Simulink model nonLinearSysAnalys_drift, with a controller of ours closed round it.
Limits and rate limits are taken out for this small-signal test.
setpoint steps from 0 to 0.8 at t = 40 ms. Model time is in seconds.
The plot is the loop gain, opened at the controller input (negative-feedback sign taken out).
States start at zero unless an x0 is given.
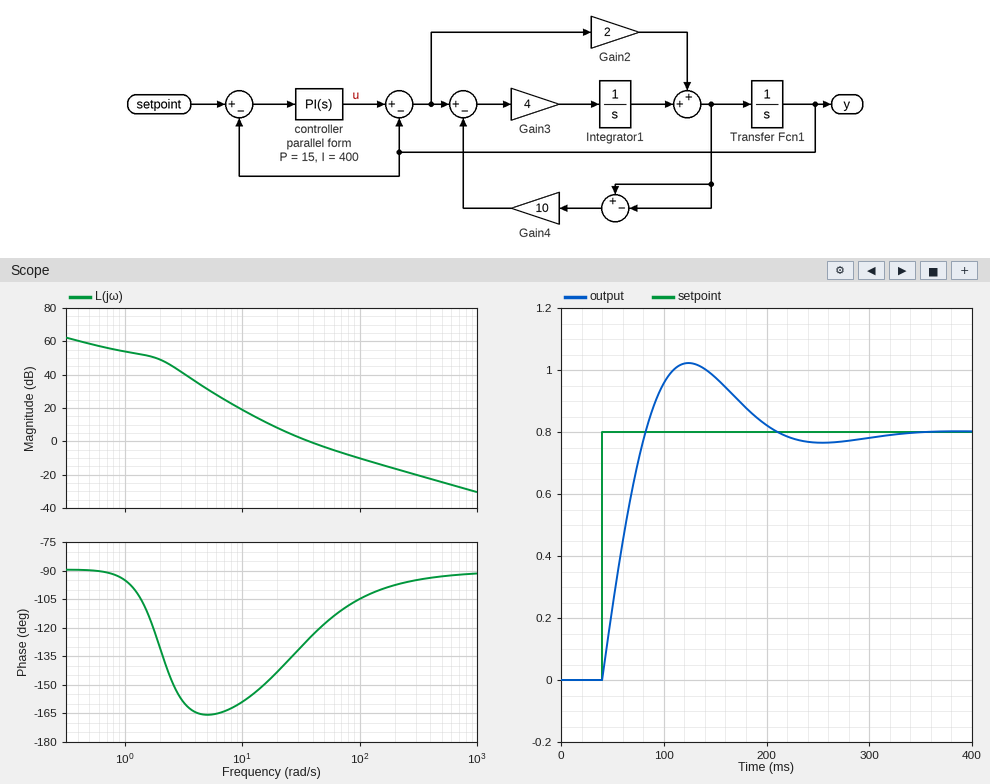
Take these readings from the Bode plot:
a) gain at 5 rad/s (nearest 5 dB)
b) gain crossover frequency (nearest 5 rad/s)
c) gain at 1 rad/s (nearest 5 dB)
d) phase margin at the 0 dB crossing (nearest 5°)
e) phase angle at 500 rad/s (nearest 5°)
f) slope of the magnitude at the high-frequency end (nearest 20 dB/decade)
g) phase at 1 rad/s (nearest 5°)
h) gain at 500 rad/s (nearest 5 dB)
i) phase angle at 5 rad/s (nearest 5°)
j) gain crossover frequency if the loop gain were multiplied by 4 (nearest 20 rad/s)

30 dB
35 rad/s
55 dB
55°
-95°
-20 dB/decade
-95°
-25 dB
-165°
120 rad/s
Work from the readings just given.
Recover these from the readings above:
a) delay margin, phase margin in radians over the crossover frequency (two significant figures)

0.027 s
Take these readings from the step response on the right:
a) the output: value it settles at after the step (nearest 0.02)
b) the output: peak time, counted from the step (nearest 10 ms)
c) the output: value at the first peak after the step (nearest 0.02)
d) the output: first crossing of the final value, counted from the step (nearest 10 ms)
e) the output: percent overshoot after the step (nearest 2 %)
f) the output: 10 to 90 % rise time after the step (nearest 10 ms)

0.80
80 ms
1.02
40 ms
28 %
30 ms
